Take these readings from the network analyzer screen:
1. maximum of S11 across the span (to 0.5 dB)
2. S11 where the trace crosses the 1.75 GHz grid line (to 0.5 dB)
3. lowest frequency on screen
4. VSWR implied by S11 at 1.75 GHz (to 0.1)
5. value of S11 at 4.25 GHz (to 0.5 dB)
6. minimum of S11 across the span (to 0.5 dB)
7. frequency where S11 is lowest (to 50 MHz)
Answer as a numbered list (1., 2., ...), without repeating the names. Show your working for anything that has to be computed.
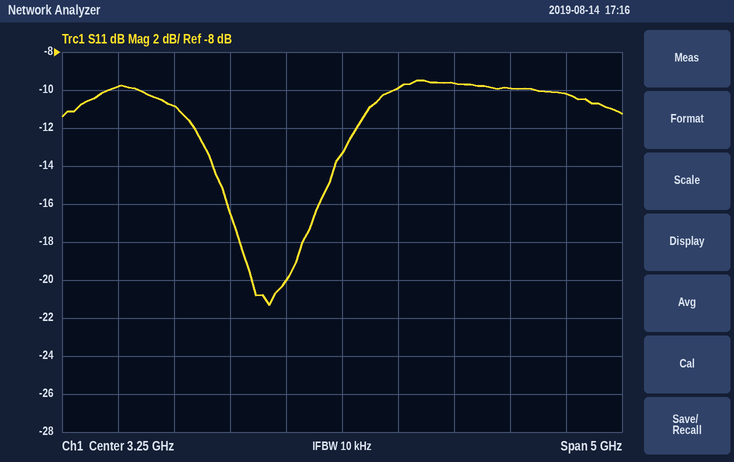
1. -9.5 dB
2. -11.0 dB
3. 750 MHz
4. |Γ| = 10^(-11/20) = 0.2818; VSWR = (1 + 0.2818)/(1 − 0.2818) ≈ 1.8
5. -9.5 dB
6. -21.5 dB
7. 2.60 GHz
